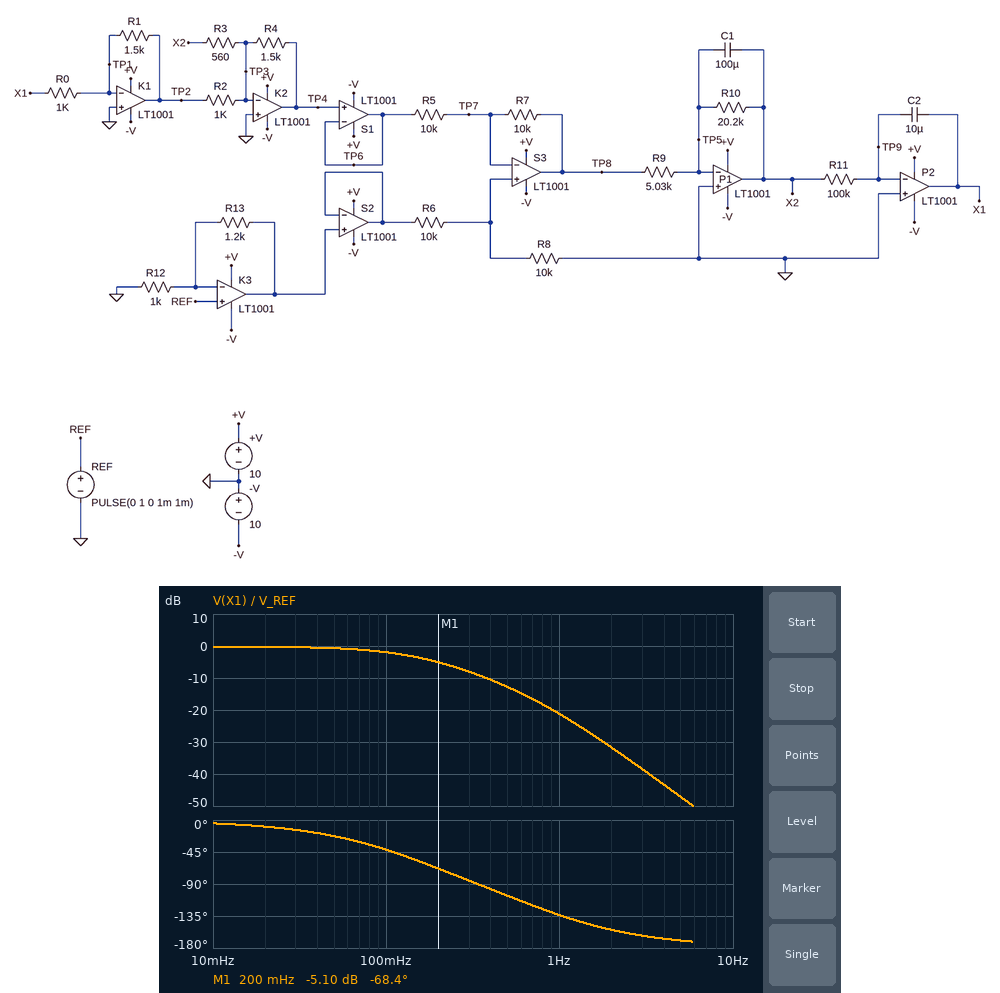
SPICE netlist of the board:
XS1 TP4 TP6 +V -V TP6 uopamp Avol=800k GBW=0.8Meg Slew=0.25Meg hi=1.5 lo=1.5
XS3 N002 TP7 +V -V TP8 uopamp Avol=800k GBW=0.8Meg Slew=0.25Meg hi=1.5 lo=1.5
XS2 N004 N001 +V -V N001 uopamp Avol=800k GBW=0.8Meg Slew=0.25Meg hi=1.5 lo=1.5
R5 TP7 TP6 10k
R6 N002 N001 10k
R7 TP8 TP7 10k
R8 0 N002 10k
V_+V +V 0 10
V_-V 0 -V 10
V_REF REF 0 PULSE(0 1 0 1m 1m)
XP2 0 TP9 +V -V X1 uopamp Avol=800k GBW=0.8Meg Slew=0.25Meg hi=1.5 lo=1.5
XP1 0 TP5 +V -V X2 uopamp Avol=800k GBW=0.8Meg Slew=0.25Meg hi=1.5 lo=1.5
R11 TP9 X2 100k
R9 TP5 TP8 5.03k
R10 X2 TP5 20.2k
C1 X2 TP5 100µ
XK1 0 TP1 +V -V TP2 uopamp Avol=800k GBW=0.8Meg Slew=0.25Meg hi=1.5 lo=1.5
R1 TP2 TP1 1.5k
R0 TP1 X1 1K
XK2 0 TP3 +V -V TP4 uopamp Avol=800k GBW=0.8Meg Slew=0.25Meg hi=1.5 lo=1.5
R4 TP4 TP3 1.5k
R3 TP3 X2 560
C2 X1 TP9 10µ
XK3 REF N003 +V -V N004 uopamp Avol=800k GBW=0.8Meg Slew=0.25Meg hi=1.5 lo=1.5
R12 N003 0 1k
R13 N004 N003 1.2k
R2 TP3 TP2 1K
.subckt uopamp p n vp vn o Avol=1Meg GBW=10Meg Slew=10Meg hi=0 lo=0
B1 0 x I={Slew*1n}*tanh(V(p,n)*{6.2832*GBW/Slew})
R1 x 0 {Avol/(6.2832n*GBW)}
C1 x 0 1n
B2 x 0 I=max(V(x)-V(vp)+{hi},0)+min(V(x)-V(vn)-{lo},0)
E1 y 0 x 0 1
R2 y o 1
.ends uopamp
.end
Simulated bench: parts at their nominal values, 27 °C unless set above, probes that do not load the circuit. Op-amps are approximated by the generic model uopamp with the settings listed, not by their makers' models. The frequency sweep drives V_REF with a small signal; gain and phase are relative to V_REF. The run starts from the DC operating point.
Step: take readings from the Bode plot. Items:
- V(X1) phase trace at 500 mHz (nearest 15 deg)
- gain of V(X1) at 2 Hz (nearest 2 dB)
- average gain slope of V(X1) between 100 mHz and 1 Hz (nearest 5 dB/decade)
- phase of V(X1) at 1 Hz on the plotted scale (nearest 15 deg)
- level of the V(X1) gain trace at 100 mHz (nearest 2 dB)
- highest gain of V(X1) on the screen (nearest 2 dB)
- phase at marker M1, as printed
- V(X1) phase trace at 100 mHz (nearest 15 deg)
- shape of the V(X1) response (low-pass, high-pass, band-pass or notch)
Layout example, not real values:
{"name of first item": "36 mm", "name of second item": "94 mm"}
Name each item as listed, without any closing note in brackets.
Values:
{"V(X1) phase trace at 500 mHz": "-105 deg", "gain of V(X1) at 2 Hz": "-32 dB", "average gain slope of V(X1) between 100 mHz and 1 Hz": "-20 dB/decade", "phase of V(X1) at 1 Hz on the plotted scale": "-135 deg", "level of the V(X1) gain trace at 100 mHz": "-2 dB", "highest gain of V(X1) on the screen": "0 dB", "phase at marker M1, as printed": "-68.4 deg", "V(X1) phase trace at 100 mHz": "-45 deg", "shape of the V(X1) response": "low-pass"}
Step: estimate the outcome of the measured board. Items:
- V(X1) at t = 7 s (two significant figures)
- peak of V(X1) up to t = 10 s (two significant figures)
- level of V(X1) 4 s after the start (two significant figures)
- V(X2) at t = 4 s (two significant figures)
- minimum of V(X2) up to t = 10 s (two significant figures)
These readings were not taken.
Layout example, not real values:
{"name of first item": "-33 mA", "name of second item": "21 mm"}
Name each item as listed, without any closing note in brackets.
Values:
{"V(X1) at t = 7 s": "980 mV", "peak of V(X1) up to t = 10 s": "980 mV", "level of V(X1) 4 s after the start": "950 mV", "V(X2) at t = 4 s": "-29 mV", "minimum of V(X2) up to t = 10 s": "-610 mV"}
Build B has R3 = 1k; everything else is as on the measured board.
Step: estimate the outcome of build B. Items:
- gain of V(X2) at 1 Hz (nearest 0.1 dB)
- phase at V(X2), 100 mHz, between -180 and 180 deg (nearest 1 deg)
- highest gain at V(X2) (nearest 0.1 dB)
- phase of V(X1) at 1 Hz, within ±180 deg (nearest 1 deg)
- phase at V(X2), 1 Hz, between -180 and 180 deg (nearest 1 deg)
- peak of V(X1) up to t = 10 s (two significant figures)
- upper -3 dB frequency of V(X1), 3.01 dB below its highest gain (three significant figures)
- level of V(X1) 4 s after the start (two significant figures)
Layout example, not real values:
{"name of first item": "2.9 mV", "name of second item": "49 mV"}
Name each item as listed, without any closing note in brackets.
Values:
{"gain of V(X2) at 1 Hz": "-3.5 dB", "phase at V(X2), 100 mHz, between -180 and 180 deg": "-118 deg", "highest gain at V(X2)": "2.0 dB", "phase of V(X1) at 1 Hz, within ±180 deg": "-148 deg", "phase at V(X2), 1 Hz, between -180 and 180 deg": "122 deg", "peak of V(X1) up to t = 10 s": "990 mV", "upper -3 dB frequency of V(X1), 3.01 dB below its highest gain": "283 mHz", "level of V(X1) 4 s after the start": "980 mV"}
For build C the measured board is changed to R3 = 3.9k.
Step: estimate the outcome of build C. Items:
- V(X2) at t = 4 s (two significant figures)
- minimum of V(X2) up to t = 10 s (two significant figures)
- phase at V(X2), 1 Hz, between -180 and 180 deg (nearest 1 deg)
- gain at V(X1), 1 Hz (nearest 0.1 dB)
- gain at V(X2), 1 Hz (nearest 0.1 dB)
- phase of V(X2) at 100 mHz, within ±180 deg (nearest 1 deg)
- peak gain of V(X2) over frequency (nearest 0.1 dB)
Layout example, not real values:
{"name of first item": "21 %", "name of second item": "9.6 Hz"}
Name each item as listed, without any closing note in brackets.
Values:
{"V(X2) at t = 4 s": "-170 mV", "minimum of V(X2) up to t = 10 s": "-1.4 V", "phase at V(X2), 1 Hz, between -180 and 180 deg": "103 deg", "gain at V(X1), 1 Hz": "-18.3 dB", "gain at V(X2), 1 Hz": "-2.3 dB", "phase of V(X2) at 100 mHz, within ±180 deg": "-101 deg", "peak gain of V(X2) over frequency": "10.8 dB"}
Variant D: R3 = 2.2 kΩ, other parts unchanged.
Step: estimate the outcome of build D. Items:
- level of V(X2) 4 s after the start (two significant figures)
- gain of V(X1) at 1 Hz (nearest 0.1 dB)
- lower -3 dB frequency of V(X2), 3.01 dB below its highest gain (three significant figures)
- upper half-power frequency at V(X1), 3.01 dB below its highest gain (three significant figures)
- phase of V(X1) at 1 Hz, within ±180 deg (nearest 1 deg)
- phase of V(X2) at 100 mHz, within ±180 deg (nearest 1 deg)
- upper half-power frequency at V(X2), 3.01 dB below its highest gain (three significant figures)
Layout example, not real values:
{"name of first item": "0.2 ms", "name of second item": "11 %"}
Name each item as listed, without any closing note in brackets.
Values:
{"level of V(X2) 4 s after the start": "-55 mV", "gain of V(X1) at 1 Hz": "-18.5 dB", "lower -3 dB frequency of V(X2), 3.01 dB below its highest gain": "220 mHz", "upper half-power frequency at V(X1), 3.01 dB below its highest gain": "399 mHz", "phase of V(X1) at 1 Hz, within ±180 deg": "-162 deg", "phase of V(X2) at 100 mHz, within ±180 deg": "-106 deg", "upper half-power frequency at V(X2), 3.01 dB below its highest gain": "515 mHz"}
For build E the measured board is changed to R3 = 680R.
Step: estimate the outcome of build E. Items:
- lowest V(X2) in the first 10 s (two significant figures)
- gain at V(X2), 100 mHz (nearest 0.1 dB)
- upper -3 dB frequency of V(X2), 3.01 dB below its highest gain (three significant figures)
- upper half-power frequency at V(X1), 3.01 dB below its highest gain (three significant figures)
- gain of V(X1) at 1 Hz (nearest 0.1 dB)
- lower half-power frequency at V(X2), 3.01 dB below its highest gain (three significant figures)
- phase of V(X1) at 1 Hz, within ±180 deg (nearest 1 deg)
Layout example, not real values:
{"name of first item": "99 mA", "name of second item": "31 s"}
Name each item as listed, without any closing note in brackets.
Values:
{"lowest V(X2) in the first 10 s": "-690 mV", "gain at V(X2), 100 mHz": "-5.4 dB", "upper -3 dB frequency of V(X2), 3.01 dB below its highest gain": "902 mHz", "upper half-power frequency at V(X1), 3.01 dB below its highest gain": "177 mHz", "gain of V(X1) at 1 Hz": "-20.5 dB", "lower half-power frequency at V(X2), 3.01 dB below its highest gain": "126 mHz", "phase of V(X1) at 1 Hz, within ±180 deg": "-139 deg"}
